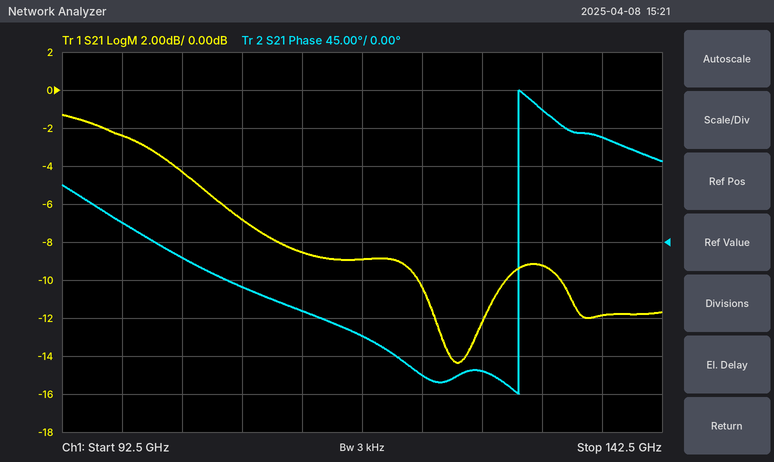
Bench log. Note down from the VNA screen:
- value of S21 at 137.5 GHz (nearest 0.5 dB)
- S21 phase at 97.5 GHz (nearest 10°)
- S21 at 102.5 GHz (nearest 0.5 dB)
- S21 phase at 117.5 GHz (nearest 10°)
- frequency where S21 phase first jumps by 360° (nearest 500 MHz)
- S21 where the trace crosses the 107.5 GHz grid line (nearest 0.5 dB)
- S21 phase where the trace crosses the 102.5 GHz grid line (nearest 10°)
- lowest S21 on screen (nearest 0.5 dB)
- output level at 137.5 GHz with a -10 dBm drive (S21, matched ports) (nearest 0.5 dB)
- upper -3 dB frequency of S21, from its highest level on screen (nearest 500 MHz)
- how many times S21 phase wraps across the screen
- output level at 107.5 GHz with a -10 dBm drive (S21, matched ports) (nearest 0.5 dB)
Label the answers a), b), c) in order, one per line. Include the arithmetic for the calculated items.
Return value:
a) -12.0 dB
b) 20°
c) -4.5 dB
d) -110°
e) 130.5 GHz
f) -7.0 dB
g) -20°
h) -14.5 dB
i) -10 dBm + (-12.0 dB) = -22.0 dBm
j) 102.5 GHz
k) 1
l) -10 dBm + (-7.0 dB) = -17.0 dBm
